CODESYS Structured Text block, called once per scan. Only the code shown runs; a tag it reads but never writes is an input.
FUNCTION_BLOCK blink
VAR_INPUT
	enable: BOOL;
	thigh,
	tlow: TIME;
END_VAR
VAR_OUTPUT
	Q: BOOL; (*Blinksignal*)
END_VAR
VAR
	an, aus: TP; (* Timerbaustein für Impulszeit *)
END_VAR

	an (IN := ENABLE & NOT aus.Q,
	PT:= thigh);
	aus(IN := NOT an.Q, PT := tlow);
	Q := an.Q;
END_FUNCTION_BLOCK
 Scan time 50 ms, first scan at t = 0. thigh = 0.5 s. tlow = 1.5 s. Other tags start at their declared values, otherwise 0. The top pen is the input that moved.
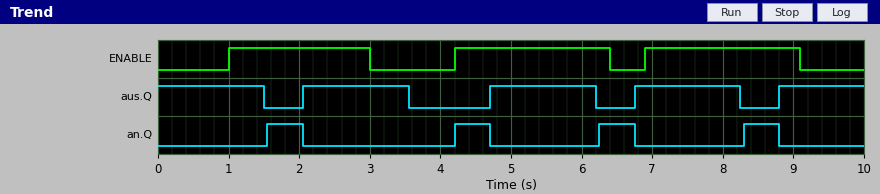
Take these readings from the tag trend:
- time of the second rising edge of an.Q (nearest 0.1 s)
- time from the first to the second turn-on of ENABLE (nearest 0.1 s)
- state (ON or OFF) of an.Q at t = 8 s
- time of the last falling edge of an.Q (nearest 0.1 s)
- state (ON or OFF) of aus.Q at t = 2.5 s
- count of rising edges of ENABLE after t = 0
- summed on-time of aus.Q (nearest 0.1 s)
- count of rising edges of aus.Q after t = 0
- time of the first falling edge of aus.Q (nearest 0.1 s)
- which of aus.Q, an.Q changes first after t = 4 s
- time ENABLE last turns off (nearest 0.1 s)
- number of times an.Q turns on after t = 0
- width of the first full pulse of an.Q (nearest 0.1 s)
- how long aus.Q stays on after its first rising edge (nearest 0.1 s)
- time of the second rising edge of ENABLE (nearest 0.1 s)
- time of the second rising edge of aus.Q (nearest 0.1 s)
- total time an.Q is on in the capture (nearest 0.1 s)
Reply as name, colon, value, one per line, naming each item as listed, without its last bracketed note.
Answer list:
time of the second rising edge of an.Q: 4.2 s
time from the first to the second turn-on of ENABLE: 3.2 s
state (ON or OFF) of an.Q at t = 8 s: OFF
time of the last falling edge of an.Q: 8.8 s
state (ON or OFF) of aus.Q at t = 2.5 s: ON
count of rising edges of ENABLE after t = 0: 3
summed on-time of aus.Q: 7.2 s
count of rising edges of aus.Q after t = 0: 4
time of the first falling edge of aus.Q: 1.5 s
which of aus.Q, an.Q changes first after t = 4 s: an.Q
time ENABLE last turns off: 9.1 s
number of times an.Q turns on after t = 0: 4
width of the first full pulse of an.Q: 0.5 s
how long aus.Q stays on after its first rising edge: 1.5 s
time of the second rising edge of ENABLE: 4.2 s
time of the second rising edge of aus.Q: 4.7 s
total time an.Q is on in the capture: 2.0 s
